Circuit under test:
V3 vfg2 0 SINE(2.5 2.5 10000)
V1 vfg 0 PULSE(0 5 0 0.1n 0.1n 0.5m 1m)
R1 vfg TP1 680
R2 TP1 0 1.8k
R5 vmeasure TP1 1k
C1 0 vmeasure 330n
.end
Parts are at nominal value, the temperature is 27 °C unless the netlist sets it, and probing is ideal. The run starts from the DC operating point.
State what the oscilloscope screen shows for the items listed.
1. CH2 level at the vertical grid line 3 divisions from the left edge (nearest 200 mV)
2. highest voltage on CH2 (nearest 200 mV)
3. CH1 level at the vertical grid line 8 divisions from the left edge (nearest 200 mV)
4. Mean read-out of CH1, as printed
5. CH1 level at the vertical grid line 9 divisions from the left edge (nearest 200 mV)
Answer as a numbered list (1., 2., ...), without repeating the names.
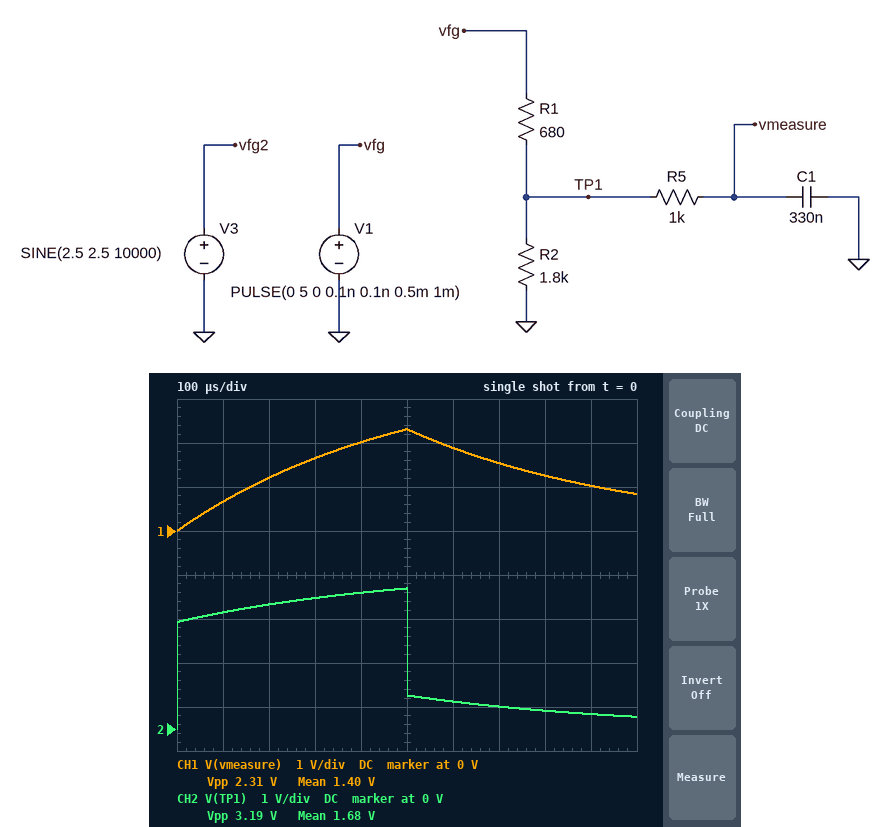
1. 3.0 V
2. 3.2 V
3. 1.2 V
4. 1.40 V
5. 1.0 V
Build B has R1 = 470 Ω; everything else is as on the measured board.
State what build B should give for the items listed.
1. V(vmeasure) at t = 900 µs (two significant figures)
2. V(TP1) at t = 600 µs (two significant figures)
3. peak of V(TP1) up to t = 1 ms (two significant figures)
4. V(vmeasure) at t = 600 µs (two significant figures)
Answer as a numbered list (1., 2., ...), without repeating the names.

1. 1.1 V
2. 580 mV
3. 3.6 V
4. 2.1 V
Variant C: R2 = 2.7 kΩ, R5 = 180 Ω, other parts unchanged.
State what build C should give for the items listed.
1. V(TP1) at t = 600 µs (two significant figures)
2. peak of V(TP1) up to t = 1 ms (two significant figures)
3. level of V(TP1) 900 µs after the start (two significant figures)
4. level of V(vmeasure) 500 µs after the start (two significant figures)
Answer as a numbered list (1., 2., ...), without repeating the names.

1. 1.7 V
2. 3.6 V
3. 490 mV
4. 3.5 V
